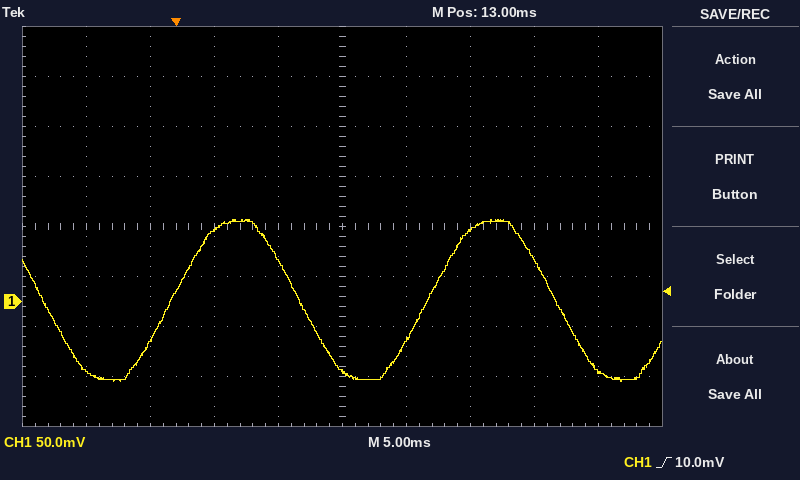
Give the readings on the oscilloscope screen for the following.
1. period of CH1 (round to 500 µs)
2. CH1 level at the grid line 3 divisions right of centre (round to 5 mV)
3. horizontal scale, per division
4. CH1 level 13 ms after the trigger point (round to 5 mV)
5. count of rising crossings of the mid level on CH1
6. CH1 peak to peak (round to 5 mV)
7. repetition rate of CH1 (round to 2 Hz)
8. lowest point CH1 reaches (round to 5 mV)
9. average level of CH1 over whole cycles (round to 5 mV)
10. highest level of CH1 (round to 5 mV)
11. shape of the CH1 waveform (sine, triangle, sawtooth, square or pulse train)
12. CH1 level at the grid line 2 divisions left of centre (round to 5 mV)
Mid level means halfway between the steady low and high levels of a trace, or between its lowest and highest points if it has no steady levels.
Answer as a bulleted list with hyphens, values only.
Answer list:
- 20.0 ms
- 40 mV
- 5 ms
- -70 mV
- 2
- 160 mV
- 50 Hz
- -80 mV
- 0 mV
- 80 mV
- sine
- 70 mV
